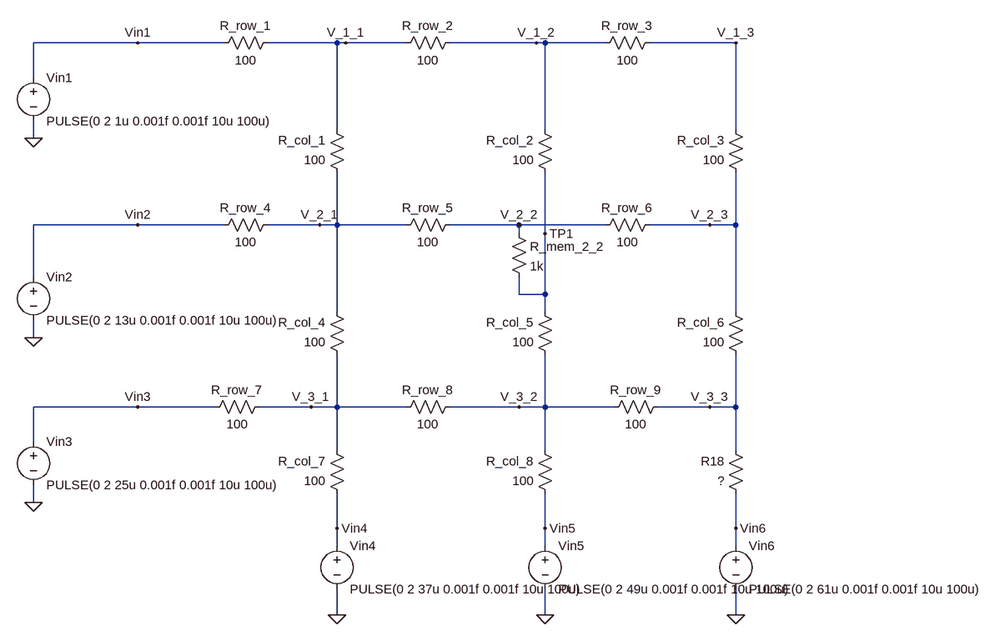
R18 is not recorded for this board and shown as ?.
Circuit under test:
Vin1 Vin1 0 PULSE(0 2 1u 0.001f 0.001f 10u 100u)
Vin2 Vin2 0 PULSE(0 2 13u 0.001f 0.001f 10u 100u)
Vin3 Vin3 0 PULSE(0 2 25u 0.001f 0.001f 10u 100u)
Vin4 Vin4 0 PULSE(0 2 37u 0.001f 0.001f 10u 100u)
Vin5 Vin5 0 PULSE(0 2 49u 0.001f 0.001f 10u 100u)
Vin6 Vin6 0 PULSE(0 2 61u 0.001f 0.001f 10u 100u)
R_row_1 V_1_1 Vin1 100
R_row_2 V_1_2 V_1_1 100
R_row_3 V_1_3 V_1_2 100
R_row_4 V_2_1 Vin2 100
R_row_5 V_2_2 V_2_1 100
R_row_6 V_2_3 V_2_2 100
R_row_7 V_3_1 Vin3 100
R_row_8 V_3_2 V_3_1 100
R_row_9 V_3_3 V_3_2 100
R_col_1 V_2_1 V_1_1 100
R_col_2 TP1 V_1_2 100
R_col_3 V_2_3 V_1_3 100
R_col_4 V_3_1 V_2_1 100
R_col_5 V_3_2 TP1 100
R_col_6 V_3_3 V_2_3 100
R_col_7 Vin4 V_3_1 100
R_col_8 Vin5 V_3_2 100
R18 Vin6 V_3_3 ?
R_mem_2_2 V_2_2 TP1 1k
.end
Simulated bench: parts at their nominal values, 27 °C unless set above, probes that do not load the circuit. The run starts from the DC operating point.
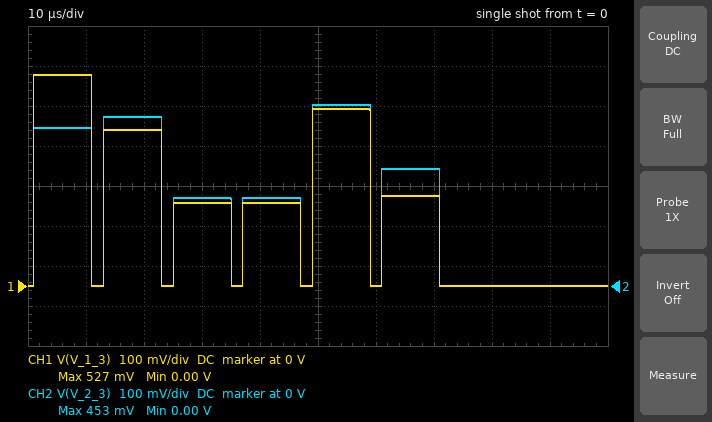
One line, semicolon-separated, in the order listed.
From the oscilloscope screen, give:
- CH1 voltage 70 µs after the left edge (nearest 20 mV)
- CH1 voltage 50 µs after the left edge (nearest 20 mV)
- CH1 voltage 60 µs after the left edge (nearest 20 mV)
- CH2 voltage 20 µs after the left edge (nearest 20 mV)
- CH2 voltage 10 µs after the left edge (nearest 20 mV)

220 mV; 440 mV; 0 V; 420 mV; 400 mV
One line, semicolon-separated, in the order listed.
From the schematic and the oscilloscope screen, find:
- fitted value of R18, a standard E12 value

330 Ω
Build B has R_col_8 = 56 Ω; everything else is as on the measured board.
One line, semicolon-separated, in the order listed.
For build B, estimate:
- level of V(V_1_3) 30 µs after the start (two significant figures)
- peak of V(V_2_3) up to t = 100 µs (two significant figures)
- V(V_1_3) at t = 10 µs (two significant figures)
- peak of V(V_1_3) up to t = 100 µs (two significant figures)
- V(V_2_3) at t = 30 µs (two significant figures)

170 mV; 600 mV; 500 mV; 590 mV; 180 mV
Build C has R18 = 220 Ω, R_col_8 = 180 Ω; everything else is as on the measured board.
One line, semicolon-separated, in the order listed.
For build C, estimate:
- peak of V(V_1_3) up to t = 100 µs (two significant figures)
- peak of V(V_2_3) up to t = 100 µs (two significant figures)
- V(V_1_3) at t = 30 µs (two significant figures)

540 mV; 430 mV; 230 mV
